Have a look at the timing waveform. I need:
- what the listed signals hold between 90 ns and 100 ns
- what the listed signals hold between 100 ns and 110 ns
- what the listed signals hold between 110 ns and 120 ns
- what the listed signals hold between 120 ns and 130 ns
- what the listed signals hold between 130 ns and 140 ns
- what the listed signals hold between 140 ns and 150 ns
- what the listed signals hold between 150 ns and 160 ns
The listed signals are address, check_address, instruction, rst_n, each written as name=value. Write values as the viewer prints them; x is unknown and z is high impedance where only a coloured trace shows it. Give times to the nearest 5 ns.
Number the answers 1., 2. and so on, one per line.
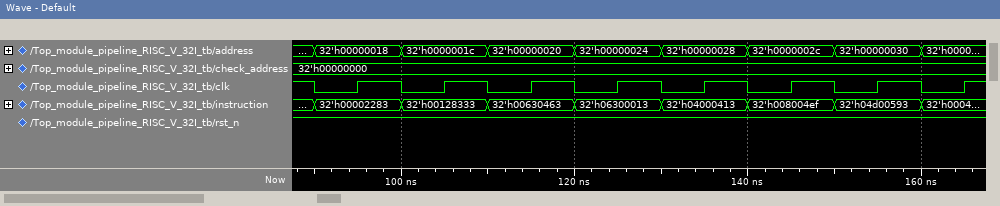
1. address=32'h00000018, check_address=32'h00000000, instruction=32'h00002283, rst_n=1
2. address=32'h0000001c, check_address=32'h00000000, instruction=32'h00128333, rst_n=1
3. address=32'h00000020, check_address=32'h00000000, instruction=32'h00630463, rst_n=1
4. address=32'h00000024, check_address=32'h00000000, instruction=32'h06300013, rst_n=1
5. address=32'h00000028, check_address=32'h00000000, instruction=32'h04000413, rst_n=1
6. address=32'h0000002c, check_address=32'h00000000, instruction=32'h008004ef, rst_n=1
7. address=32'h00000030, check_address=32'h00000000, instruction=32'h04d00593, rst_n=1
